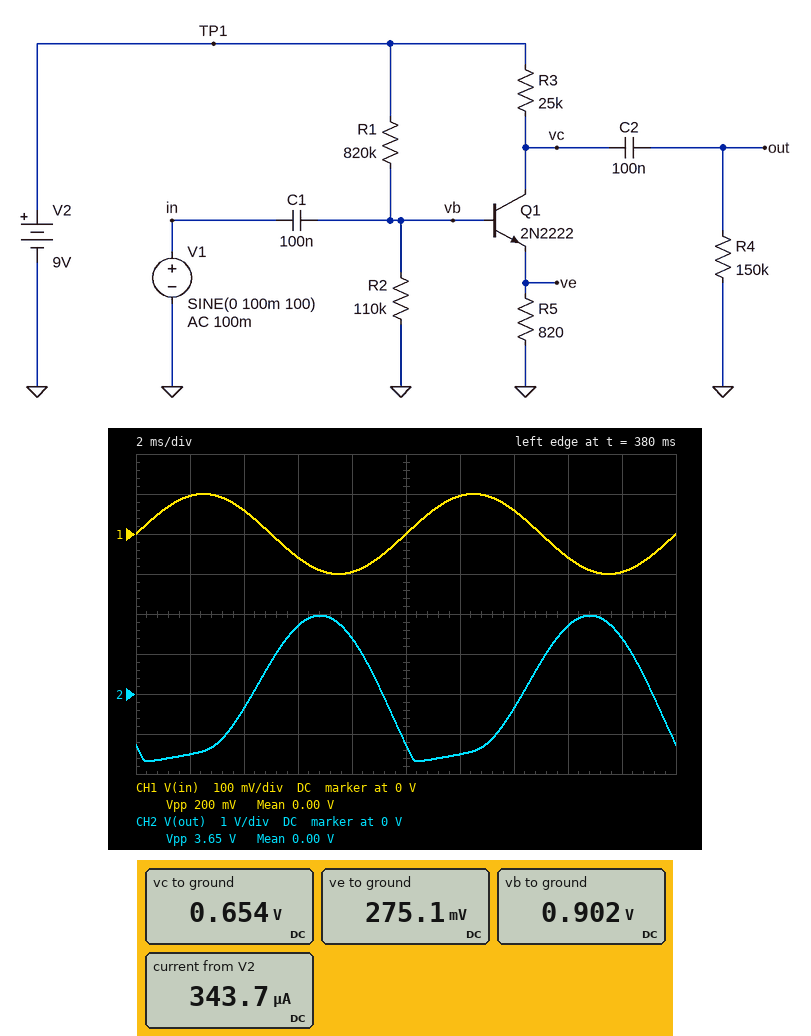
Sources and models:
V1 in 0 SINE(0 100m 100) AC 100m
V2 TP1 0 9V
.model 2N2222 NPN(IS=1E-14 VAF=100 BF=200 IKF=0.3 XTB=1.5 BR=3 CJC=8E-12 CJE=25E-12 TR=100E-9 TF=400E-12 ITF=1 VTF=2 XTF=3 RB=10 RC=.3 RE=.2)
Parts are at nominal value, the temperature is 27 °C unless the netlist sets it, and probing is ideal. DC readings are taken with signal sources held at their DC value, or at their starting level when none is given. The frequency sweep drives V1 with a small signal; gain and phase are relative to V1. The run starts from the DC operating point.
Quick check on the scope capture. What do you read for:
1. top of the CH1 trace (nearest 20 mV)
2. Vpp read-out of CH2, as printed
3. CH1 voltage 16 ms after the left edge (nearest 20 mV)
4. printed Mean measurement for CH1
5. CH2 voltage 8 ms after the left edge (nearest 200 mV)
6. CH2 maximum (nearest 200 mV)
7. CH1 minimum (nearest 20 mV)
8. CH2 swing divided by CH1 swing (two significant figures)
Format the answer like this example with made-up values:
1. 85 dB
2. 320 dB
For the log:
1. 100 mV
2. 3.65 V
3. -60 mV
4. 0.00 V
5. 1.4 V
6. 2.0 V
7. -100 mV
8. 18
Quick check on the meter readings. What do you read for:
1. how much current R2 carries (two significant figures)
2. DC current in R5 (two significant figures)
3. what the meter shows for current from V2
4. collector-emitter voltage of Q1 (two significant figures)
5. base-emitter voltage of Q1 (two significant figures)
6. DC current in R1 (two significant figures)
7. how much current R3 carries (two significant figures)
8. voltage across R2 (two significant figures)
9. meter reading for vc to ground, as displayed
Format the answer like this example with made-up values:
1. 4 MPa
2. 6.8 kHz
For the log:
1. 8.2 µA
2. 340 µA
3. 343.7 µA
4. 380 mV
5. 630 mV
6. 9.9 µA
7. 330 µA
8. 900 mV
9. 0.654 V
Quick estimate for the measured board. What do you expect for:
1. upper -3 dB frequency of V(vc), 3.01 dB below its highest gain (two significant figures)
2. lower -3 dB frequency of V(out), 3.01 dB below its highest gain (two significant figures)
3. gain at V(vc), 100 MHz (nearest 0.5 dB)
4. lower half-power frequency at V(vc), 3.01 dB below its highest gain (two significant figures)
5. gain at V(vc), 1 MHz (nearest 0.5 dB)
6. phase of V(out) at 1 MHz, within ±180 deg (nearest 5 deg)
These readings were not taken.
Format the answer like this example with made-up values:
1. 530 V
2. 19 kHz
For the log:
1. 810 kHz
2. 29 Hz
3. 0.5 dB
4. 25 Hz
5. 23.5 dB
6. 125 deg
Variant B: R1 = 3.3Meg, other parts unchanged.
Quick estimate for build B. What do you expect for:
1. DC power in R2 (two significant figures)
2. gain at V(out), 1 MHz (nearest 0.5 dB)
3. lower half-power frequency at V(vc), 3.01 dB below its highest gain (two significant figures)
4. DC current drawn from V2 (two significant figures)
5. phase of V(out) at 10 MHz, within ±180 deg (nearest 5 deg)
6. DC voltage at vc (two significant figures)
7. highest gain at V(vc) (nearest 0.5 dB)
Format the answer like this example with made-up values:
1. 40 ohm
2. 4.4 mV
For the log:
1. 770 nW
2. -7.5 dB
3. 2.1 MHz
4. 2.6 µA
5. 10 deg
6. 9.0 V
7. 0 dB
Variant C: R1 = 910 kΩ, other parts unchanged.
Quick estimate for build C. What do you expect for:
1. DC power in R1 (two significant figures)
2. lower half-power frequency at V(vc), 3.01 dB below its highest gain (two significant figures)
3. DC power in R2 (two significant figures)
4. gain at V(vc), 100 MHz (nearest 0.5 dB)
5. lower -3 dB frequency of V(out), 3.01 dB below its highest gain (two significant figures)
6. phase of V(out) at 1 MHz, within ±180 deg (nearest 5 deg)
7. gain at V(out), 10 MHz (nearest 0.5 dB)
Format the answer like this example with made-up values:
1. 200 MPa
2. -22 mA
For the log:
1. 73 µW
2. 24 Hz
3. 6.4 µW
4. 1.0 dB
5. 28 Hz
6. 140 deg
7. 10.5 dB
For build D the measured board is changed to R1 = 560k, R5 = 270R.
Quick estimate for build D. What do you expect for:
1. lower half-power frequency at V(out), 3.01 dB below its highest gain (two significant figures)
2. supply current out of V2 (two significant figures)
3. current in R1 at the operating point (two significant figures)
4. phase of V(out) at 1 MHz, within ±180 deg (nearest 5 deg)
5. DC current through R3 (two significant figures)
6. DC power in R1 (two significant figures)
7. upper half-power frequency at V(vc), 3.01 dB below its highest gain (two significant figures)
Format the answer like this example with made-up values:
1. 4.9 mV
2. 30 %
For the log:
1. 2.6 kHz
2. 370 µA
3. 15 µA
4. 115 deg
5. 350 µA
6. 120 µW
7. 840 kHz
